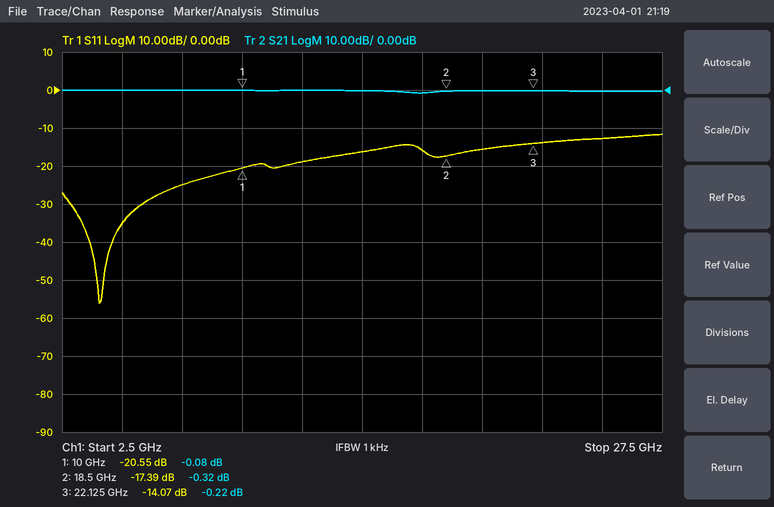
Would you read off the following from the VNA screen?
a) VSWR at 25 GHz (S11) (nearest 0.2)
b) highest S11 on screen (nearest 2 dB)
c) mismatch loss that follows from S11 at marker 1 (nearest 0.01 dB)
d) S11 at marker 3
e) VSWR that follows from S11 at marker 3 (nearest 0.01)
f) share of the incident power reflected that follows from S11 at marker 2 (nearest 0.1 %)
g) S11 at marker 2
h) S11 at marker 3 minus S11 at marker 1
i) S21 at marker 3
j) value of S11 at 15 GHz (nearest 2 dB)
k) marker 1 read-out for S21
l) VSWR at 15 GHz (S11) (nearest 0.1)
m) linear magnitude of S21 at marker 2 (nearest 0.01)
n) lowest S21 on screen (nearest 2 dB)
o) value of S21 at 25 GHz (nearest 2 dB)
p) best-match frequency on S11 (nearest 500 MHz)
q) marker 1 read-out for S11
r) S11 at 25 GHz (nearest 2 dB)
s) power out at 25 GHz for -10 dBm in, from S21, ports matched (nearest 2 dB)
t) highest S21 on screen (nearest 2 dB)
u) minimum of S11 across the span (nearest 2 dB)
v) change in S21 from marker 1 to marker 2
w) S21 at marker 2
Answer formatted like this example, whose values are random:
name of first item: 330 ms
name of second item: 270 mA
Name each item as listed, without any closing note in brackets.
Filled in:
VSWR at 25 GHz (S11): 1.6
highest S11 on screen: -12 dB
mismatch loss that follows from S11 at marker 1: 0.04 dB
S11 at marker 3: -14.07 dB
VSWR that follows from S11 at marker 3: 1.49
share of the incident power reflected that follows from S11 at marker 2: 1.8 %
S11 at marker 2: -17.39 dB
S11 at marker 3 minus S11 at marker 1: 6.48 dB
S21 at marker 3: -0.22 dB
value of S11 at 15 GHz: -16 dB
marker 1 read-out for S21: -0.08 dB
VSWR at 15 GHz (S11): 1.4
linear magnitude of S21 at marker 2: 0.96
lowest S21 on screen: 0 dB
value of S21 at 25 GHz: 0 dB
best-match frequency on S11: 4.0 GHz
marker 1 read-out for S11: -20.55 dB
S11 at 25 GHz: -12 dB
power out at 25 GHz for -10 dBm in, from S21, ports matched: -10 dBm
highest S21 on screen: 0 dB
minimum of S11 across the span: -56 dB
change in S21 from marker 1 to marker 2: -0.24 dB
S21 at marker 2: -0.32 dB
